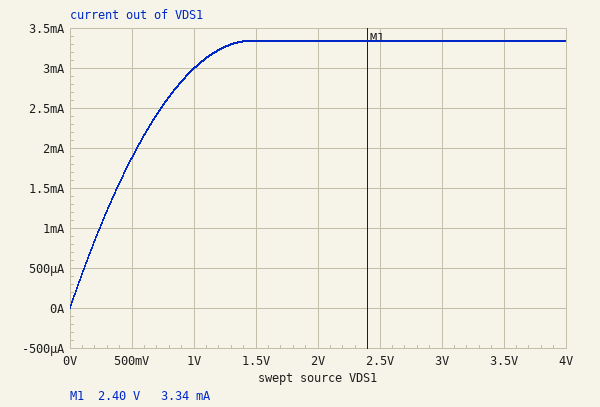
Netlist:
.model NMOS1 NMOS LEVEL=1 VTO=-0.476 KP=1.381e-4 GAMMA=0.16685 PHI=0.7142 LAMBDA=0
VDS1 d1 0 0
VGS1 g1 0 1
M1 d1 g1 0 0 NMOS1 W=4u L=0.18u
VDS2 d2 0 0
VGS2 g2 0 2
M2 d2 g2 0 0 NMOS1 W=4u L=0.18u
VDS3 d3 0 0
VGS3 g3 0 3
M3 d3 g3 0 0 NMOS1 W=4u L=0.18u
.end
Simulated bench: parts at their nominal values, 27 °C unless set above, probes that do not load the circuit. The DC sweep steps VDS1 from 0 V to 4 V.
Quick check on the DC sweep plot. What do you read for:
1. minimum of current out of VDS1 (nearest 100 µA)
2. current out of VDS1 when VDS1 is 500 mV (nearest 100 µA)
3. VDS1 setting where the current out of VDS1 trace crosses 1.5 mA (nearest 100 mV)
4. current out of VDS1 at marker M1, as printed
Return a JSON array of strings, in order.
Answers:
["0 A", "1.9 mA", "400 mV", "3.34 mA"]
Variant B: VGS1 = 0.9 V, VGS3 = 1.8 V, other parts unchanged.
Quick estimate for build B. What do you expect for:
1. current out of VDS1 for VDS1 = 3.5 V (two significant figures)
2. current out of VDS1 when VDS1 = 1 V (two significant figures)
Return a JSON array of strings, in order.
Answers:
["2.9 mA", "2.7 mA"]
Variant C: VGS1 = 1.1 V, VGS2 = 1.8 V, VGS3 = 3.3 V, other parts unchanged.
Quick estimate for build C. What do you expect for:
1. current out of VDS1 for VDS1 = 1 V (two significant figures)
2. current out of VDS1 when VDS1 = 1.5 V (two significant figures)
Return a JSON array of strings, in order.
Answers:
["3.3 mA", "3.8 mA"]
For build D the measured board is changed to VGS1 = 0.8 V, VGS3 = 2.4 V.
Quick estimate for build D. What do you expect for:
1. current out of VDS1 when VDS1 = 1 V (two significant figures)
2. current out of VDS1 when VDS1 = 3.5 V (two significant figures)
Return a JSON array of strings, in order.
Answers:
["2.4 mA", "2.5 mA"]
